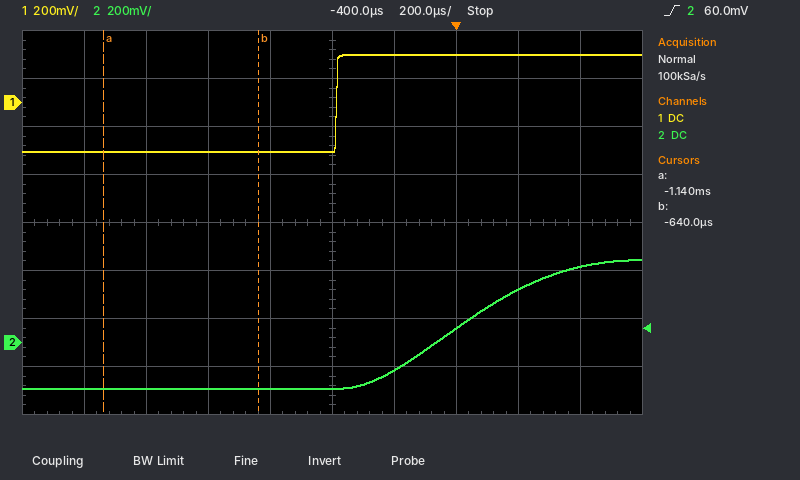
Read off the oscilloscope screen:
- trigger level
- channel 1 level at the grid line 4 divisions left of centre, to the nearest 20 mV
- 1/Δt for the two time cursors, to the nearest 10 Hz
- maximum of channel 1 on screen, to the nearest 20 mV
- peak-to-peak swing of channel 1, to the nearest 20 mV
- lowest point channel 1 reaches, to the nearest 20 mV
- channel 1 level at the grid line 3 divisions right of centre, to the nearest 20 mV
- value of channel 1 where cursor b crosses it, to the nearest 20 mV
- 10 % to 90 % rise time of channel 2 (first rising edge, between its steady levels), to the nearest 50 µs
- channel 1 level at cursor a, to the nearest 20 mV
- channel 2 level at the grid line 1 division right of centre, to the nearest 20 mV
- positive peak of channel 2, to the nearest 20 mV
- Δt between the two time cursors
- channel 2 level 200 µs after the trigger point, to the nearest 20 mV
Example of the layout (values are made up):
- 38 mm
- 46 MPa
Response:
- 60.0 mV
- -200 mV
- 2.00 kHz
- 200 mV
- 400 mV
- -200 mV
- 200 mV
- -200 mV
- 550 µs
- -200 mV
- -120 mV
- 340 mV
- 500 µs
- 220 mV
